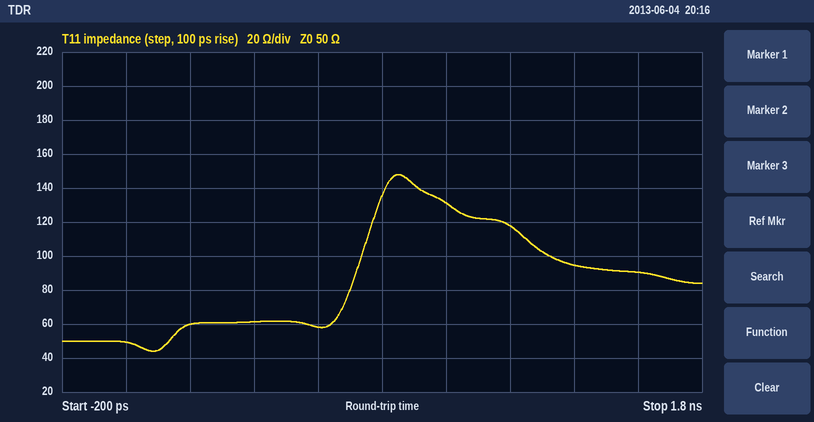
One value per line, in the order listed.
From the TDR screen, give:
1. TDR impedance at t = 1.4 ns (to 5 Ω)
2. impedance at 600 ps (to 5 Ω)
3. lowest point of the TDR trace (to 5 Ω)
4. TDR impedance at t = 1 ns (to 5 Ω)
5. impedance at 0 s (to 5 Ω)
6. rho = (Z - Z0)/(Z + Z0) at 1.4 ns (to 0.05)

95 Ω
60 Ω
45 Ω
130 Ω
50 Ω
+0.30
